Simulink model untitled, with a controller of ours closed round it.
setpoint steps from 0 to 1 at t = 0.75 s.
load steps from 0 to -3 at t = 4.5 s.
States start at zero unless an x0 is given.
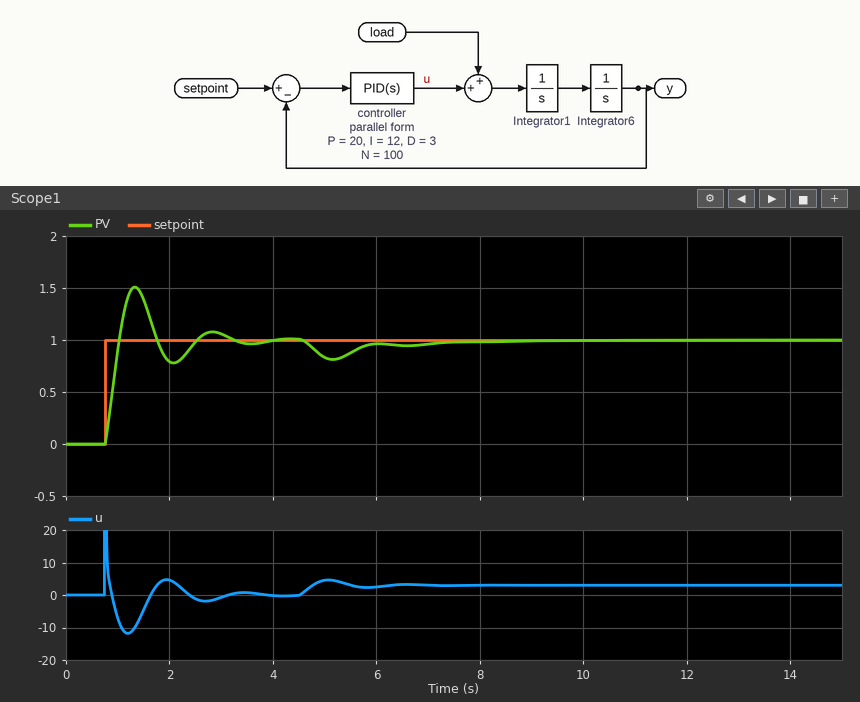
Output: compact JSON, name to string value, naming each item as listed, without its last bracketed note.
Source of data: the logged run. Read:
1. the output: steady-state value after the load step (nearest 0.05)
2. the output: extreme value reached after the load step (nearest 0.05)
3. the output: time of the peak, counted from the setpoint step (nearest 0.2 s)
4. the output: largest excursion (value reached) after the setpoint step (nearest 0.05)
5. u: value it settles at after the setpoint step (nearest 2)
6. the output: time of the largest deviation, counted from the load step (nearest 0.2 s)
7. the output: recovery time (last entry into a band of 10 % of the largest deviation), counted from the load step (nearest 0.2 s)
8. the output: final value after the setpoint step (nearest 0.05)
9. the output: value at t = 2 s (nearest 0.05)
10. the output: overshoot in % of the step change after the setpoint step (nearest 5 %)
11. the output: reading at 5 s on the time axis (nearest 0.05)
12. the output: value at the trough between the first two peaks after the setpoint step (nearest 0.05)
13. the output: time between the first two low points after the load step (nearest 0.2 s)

{"the output: steady-state value after the load step": "1.00", "the output: extreme value reached after the load step": "0.80", "the output: time of the peak, counted from the setpoint step": "0.6 s", "the output: largest excursion (value reached) after the setpoint step": "1.50", "u: value it settles at after the setpoint step": "0", "the output: time of the largest deviation, counted from the load step": "0.6 s", "the output: recovery time (last entry into a band of 10 % of the largest deviation), counted from the load step": "3.0 s", "the output: final value after the setpoint step": "1.00", "the output: value at t = 2 s": "0.80", "the output: overshoot in % of the step change after the setpoint step": "50 %", "the output: reading at 5 s on the time axis": "0.85", "the output: value at the trough between the first two peaks after the setpoint step": "0.80", "the output: time between the first two low points after the load step": "1.4 s"}
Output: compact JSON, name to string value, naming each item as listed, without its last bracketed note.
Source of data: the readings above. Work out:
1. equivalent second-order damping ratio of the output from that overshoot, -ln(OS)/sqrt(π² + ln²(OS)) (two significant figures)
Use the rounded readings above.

{"equivalent second-order damping ratio of the output from that overshoot, -ln(OS)/sqrt(π² + ln²(OS))": "0.22"}
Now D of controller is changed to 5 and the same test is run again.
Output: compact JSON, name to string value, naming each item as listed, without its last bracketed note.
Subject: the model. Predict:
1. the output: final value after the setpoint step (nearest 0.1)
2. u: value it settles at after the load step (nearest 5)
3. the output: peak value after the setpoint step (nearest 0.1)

{"the output: final value after the setpoint step": "1.0", "u: value it settles at after the load step": "5", "the output: peak value after the setpoint step": "1.3"}
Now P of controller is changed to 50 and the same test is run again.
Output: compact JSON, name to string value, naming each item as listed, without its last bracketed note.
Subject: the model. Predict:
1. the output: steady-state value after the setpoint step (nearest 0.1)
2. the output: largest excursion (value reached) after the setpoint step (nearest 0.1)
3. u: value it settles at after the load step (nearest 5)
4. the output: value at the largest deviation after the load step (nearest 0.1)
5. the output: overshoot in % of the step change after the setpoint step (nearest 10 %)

{"the output: steady-state value after the setpoint step": "1.0", "the output: largest excursion (value reached) after the setpoint step": "1.6", "u: value it settles at after the load step": "5", "the output: value at the largest deviation after the load step": "0.9", "the output: overshoot in % of the step change after the setpoint step": "60 %"}
